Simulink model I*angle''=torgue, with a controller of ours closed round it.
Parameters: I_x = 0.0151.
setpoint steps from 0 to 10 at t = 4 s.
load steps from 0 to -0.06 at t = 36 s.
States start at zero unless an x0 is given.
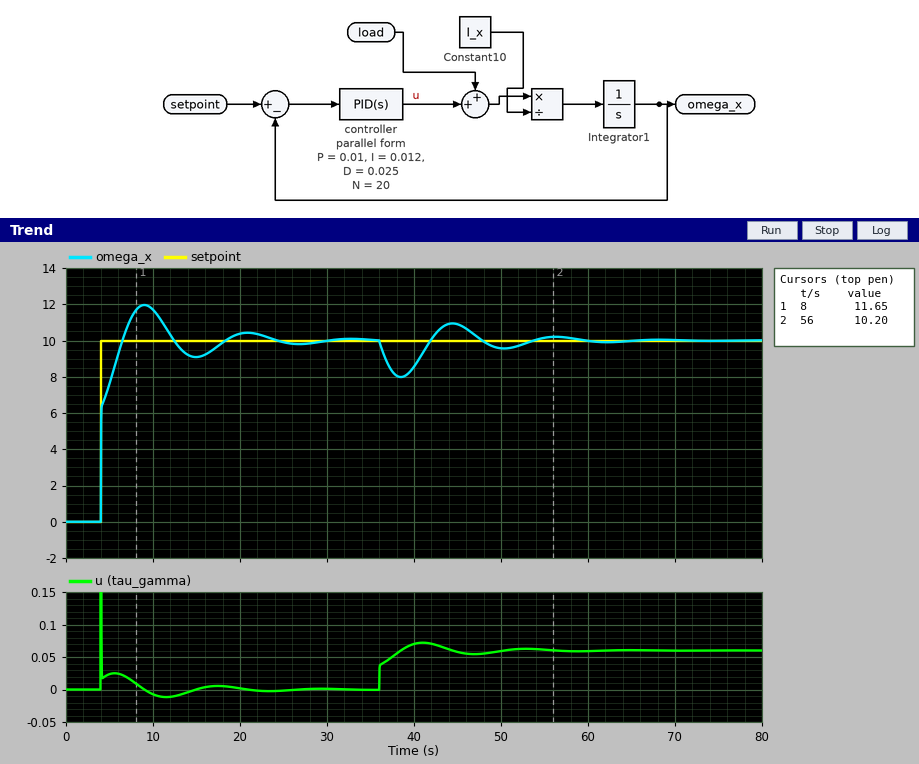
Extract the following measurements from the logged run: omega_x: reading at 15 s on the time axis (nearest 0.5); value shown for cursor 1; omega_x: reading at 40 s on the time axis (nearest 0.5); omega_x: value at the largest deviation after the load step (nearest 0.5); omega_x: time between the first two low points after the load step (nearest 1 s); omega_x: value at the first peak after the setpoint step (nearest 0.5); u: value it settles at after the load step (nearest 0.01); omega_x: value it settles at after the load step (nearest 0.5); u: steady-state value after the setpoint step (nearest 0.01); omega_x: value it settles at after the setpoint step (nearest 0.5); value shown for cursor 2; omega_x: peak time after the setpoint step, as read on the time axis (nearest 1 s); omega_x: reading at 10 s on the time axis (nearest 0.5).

9.0
11.65
8.5
8.0
12 s
12.0
0.06
10.0
0.00
10.0
10.20
9 s
11.5
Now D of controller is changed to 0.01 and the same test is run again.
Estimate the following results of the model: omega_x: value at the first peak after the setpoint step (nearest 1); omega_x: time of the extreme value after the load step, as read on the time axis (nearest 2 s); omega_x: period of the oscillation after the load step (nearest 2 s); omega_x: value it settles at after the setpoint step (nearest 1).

13
38 s
10 s
10
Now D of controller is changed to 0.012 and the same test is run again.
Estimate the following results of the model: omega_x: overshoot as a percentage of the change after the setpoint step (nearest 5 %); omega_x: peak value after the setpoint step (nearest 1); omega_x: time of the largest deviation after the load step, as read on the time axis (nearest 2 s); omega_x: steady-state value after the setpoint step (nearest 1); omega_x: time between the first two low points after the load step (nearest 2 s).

25 %
13
38 s
10
10 s
